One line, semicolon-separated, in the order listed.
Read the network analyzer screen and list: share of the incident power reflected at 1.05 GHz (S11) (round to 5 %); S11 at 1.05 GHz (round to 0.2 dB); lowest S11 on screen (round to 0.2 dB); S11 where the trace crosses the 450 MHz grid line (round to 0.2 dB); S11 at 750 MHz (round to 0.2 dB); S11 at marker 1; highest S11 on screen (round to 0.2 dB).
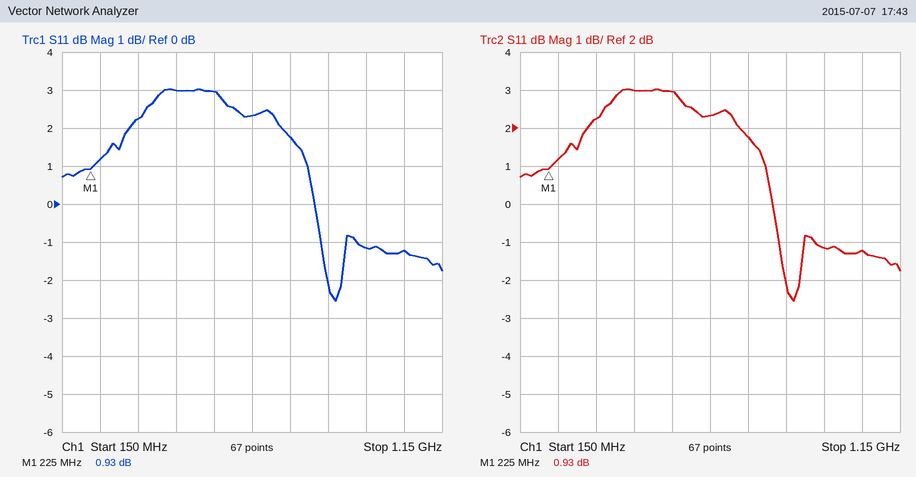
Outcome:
75 %; -1.2 dB; -2.6 dB; 3.0 dB; 1.8 dB; 0.93 dB; 3.0 dB
